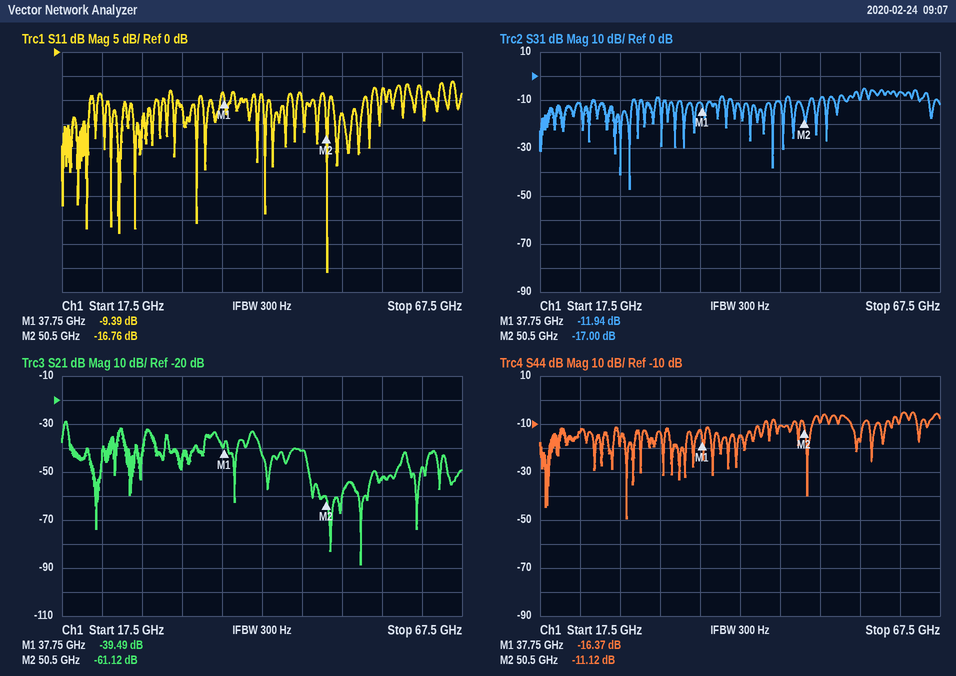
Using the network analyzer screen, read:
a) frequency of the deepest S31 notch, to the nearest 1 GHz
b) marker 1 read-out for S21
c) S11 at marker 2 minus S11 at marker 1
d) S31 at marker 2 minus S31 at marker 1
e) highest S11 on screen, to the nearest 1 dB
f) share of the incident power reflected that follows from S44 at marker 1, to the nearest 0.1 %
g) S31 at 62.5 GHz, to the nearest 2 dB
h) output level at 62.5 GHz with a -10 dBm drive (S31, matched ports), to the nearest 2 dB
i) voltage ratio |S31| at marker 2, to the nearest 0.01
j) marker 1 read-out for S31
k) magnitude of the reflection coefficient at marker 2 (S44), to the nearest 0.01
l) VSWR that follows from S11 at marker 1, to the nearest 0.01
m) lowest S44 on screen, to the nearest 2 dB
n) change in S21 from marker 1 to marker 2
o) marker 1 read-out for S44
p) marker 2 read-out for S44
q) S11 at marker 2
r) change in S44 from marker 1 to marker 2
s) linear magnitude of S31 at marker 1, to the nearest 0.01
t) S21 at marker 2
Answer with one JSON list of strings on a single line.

["29 GHz", "-39.49 dB", "-7.37 dB", "-5.06 dB", "-6 dB", "2.3 %", "-6 dB", "-16 dBm", "0.14", "-11.94 dB", "0.28", "2.03", "-50 dB", "-21.63 dB", "-16.37 dB", "-11.12 dB", "-16.76 dB", "5.25 dB", "0.25", "-61.12 dB"]
